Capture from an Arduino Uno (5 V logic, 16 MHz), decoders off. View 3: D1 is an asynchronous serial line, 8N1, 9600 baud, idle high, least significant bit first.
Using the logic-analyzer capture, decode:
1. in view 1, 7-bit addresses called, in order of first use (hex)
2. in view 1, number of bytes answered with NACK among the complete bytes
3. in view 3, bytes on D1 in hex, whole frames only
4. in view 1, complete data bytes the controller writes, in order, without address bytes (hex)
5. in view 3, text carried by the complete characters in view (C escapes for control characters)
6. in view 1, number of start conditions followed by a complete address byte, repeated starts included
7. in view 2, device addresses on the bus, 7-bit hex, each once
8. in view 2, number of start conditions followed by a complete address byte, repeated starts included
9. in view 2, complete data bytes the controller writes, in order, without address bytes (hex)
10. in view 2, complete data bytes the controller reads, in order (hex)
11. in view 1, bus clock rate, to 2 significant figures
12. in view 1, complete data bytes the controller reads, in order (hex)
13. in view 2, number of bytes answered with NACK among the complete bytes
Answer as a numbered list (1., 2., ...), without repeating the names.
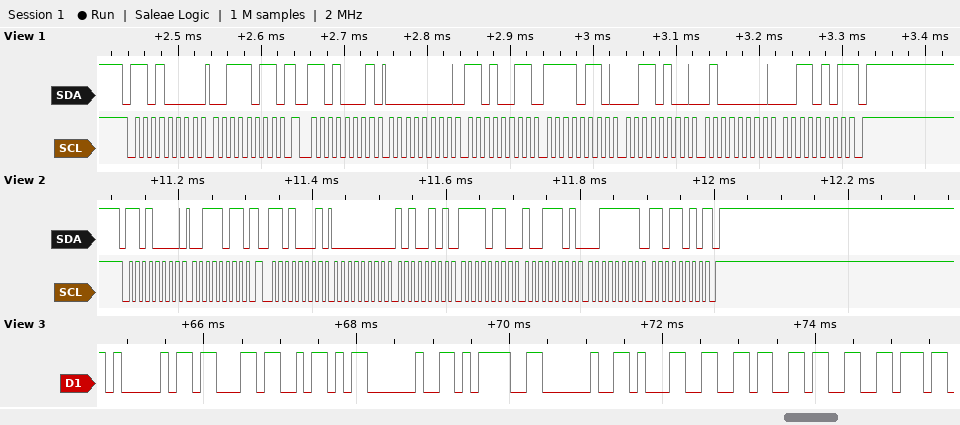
1. 0x68
2. 1
3. 41 63 5A 20 3D 20 31 36 33
4. 3B
5. "AcZ = 163"
6. 2
7. 0x68
8. 2
9. 3B
10. 00 A5 F6 9D 3F DA
11. 100 kHz
12. 00 D3 F6 34 40 35
13. 1
